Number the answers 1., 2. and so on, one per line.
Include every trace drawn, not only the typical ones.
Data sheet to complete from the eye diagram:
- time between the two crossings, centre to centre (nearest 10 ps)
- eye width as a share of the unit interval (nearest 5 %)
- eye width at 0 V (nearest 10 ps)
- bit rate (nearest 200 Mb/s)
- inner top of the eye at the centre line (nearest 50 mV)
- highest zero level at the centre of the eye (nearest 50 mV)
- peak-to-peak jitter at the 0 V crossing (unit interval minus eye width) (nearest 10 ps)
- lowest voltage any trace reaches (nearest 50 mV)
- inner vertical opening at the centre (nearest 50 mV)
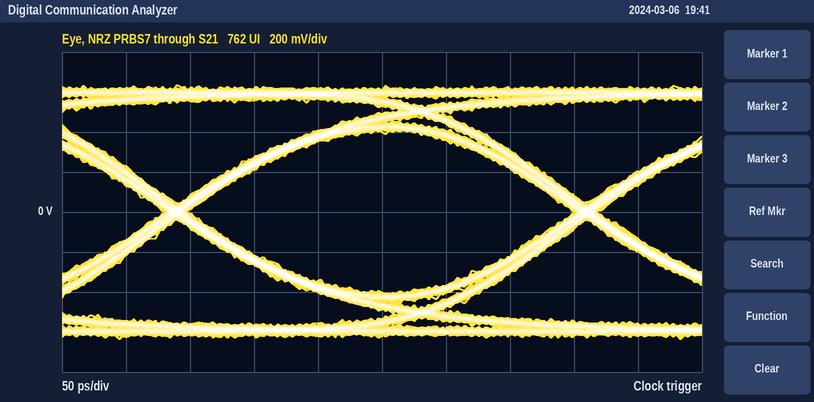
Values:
1. 320 ps
2. 95 %
3. 300 ps
4. 3.2 Gb/s
5. 400 mV
6. -400 mV
7. 20 ps
8. -650 mV
9. 800 mV
